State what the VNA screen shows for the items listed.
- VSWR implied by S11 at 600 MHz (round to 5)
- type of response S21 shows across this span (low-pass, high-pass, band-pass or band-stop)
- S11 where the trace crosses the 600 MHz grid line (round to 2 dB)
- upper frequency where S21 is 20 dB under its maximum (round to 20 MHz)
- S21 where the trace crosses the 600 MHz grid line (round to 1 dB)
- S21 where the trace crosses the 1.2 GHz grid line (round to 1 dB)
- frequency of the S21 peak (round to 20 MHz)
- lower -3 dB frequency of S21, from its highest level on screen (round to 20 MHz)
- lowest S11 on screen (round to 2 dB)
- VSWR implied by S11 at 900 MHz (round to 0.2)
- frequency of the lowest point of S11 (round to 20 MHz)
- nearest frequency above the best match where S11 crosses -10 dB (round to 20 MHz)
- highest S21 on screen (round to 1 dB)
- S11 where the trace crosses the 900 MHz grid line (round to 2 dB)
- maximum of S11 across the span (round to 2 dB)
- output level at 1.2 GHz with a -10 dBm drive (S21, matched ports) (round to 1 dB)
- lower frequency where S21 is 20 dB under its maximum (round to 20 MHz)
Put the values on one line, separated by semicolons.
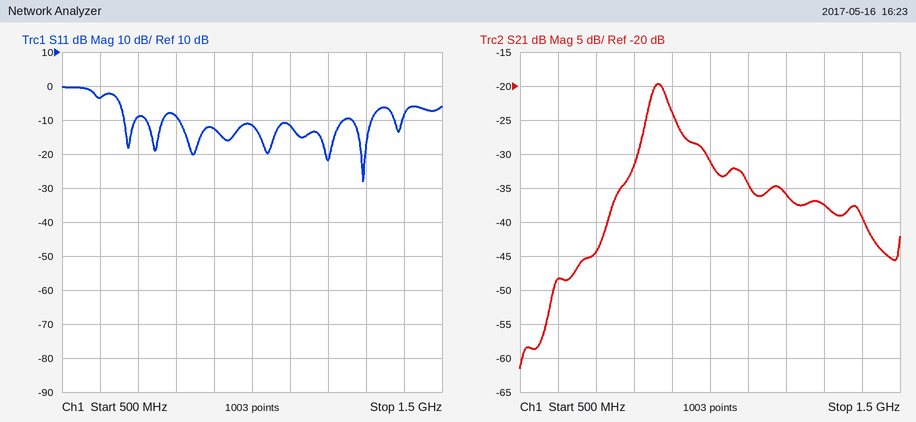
5; band-pass; -4 dB; 1.40 GHz; -48 dB; -36 dB; 860 MHz; 840 MHz; -28 dB; 1.6; 1.30 GHz; 1.32 GHz; -20 dB; -12 dB; 0 dB; -46 dBm; 740 MHz
